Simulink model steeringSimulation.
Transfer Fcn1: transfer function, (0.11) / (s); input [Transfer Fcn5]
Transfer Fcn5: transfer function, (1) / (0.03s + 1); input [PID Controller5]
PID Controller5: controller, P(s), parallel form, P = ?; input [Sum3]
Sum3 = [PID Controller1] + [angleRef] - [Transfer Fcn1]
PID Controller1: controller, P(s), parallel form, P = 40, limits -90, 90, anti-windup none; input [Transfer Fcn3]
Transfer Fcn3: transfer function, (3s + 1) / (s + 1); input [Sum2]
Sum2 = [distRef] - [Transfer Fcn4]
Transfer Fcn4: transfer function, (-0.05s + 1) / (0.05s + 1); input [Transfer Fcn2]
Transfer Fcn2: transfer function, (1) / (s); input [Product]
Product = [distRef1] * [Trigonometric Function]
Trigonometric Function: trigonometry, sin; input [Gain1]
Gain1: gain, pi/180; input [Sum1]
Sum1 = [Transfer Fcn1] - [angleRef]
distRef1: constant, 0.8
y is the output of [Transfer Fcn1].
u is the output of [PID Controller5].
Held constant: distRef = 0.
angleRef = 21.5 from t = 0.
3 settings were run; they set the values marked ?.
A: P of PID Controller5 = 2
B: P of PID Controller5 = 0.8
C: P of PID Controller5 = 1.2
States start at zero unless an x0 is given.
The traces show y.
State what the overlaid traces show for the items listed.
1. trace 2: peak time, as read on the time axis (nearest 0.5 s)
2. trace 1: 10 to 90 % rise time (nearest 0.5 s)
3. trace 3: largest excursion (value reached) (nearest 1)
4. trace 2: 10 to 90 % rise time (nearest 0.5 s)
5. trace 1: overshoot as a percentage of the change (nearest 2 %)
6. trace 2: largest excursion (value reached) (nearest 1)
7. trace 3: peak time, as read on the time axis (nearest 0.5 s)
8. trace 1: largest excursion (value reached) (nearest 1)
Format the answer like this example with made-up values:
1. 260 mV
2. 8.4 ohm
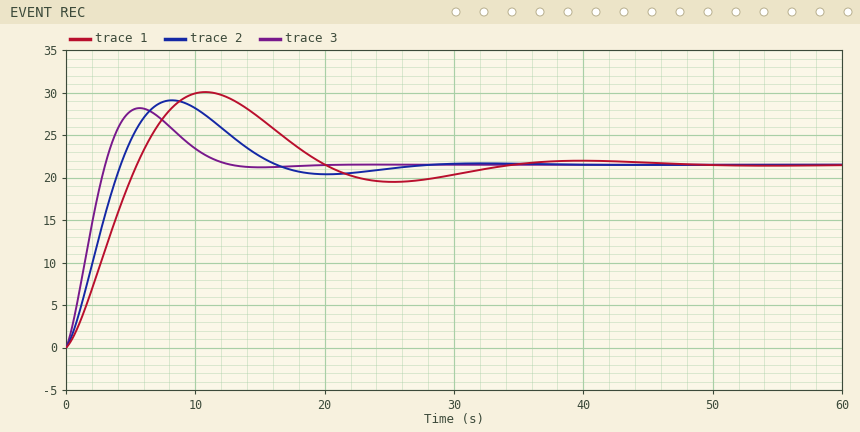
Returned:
1. 8.0 s
2. 4.0 s
3. 28
4. 3.0 s
5. 40 %
6. 29
7. 5.5 s
8. 30
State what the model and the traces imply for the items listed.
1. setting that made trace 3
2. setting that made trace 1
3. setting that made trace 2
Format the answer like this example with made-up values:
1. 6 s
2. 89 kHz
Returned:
1. A
2. B
3. C
